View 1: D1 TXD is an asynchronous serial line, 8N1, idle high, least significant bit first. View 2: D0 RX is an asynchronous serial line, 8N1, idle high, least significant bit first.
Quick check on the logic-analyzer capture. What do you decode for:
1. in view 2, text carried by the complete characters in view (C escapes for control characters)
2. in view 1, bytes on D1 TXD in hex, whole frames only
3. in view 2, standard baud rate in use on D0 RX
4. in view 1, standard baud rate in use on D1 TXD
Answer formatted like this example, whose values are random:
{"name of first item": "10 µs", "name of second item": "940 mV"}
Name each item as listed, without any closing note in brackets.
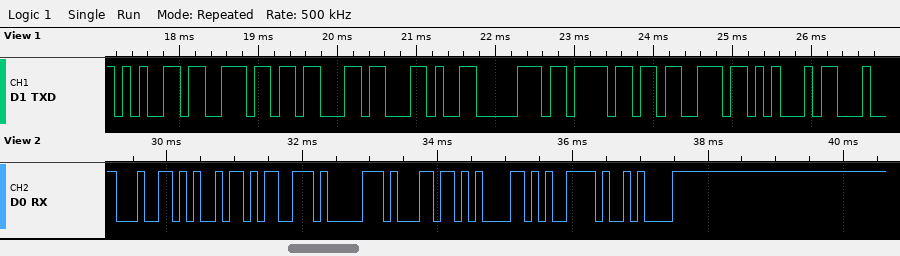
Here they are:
{"in view 2, text carried by the complete characters in view": "\"display\\n\"", "in view 1, bytes on D1 TXD in hex, whole frames only": "65 6E 63 2C 70 6F 73 45", "in view 2, standard baud rate in use on D0 RX": "9600 baud", "in view 1, standard baud rate in use on D1 TXD": "9600 baud"}
